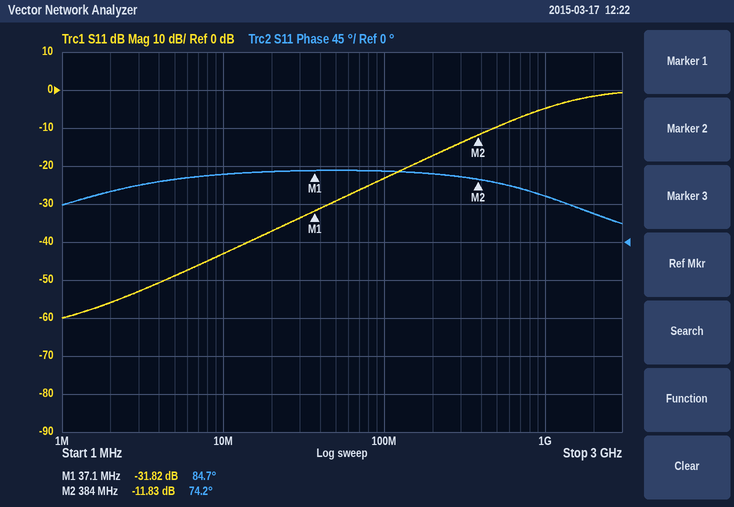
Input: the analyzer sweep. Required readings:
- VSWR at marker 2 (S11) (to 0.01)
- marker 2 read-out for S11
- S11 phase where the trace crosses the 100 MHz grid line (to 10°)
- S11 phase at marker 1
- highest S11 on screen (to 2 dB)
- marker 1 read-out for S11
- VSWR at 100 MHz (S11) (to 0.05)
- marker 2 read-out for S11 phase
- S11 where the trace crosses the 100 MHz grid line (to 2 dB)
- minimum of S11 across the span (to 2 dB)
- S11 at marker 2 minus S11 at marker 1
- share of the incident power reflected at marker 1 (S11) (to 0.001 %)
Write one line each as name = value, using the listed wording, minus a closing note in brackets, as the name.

VSWR at marker 2 (S11) = 1.69
marker 2 read-out for S11 = -11.83 dB
S11 phase where the trace crosses the 100 MHz grid line = 80°
S11 phase at marker 1 = 84.7°
highest S11 on screen = 0 dB
marker 1 read-out for S11 = -31.82 dB
VSWR at 100 MHz (S11) = 1.15
marker 2 read-out for S11 phase = 74.2°
S11 where the trace crosses the 100 MHz grid line = -24 dB
minimum of S11 across the span = -60 dB
S11 at marker 2 minus S11 at marker 1 = 19.99 dB
share of the incident power reflected at marker 1 (S11) = 0.066 %
